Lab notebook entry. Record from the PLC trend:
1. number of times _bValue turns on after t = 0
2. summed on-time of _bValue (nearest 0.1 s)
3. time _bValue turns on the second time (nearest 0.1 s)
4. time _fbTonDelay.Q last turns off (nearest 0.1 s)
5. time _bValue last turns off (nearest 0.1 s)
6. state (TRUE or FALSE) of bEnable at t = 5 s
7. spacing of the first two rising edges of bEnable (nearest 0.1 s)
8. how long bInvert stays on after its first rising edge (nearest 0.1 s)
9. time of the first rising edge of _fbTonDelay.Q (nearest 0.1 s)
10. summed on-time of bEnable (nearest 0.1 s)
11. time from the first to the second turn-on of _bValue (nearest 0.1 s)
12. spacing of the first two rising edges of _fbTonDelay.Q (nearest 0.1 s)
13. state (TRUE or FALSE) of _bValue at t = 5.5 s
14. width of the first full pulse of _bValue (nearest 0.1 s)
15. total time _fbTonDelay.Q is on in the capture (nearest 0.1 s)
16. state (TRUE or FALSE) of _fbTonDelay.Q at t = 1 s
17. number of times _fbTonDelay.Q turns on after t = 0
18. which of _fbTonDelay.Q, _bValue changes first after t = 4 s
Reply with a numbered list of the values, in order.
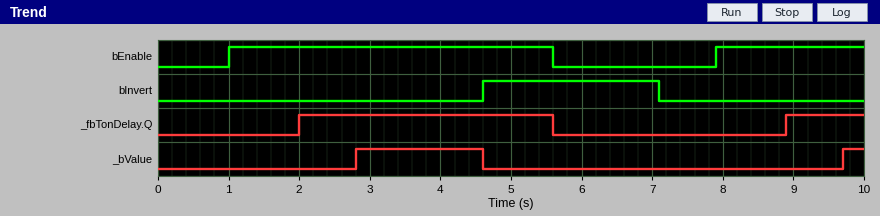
1. 2
2. 2.1 s
3. 9.7 s
4. 5.6 s
5. 4.6 s
6. TRUE
7. 6.9 s
8. 2.5 s
9. 2.0 s
10. 6.7 s
11. 6.9 s
12. 6.9 s
13. FALSE
14. 1.8 s
15. 4.7 s
16. FALSE
17. 2
18. _bValue
